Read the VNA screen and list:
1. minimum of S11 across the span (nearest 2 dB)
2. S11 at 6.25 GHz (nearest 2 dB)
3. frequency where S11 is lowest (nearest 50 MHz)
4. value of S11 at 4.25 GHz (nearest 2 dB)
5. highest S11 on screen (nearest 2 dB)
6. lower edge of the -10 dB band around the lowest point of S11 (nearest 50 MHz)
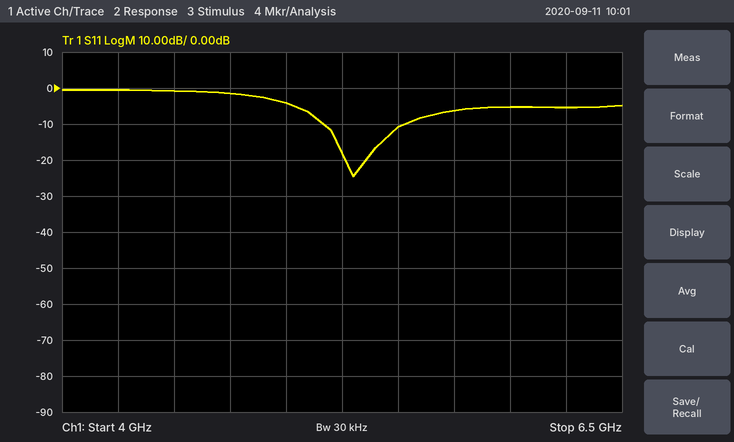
-24 dB
-6 dB
5.30 GHz
0 dB
0 dB
5.15 GHz
